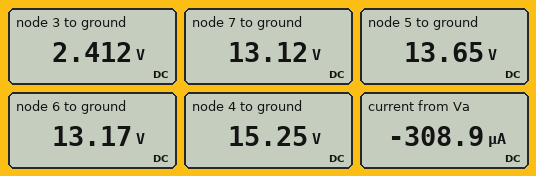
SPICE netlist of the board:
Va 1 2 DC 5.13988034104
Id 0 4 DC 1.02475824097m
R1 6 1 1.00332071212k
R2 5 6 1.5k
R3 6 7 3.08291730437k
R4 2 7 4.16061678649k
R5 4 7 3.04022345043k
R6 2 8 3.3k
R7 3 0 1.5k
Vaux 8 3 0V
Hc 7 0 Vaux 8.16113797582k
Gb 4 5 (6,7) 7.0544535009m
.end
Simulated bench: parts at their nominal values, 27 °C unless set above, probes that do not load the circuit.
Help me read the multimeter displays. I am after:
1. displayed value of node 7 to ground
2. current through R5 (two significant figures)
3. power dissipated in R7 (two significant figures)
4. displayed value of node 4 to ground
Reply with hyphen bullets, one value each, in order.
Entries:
- 13.12 V
- 700 µA
- 3.9 mW
- 15.25 V
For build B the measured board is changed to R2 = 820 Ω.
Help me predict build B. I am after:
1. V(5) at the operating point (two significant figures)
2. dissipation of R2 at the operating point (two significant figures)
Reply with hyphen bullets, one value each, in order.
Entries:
- 13 V
- 86 µW
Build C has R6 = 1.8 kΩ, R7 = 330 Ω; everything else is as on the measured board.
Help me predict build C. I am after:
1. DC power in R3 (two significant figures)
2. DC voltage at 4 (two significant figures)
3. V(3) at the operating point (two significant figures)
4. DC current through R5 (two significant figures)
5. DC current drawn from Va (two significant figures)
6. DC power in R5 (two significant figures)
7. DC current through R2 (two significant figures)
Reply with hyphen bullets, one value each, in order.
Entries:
- 930 nW
- 11 V
- 260 mV
- 1.4 mA
- 360 µA
- 6.0 mW
- 380 µA
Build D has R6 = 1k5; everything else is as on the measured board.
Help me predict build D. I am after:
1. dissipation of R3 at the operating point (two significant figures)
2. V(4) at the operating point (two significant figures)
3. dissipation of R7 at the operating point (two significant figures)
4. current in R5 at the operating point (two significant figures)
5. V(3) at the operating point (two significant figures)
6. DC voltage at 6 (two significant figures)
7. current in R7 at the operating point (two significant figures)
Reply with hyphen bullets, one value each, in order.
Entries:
- 380 nW
- 12 V
- 1.4 mW
- 1.3 mA
- 1.4 V
- 7.8 V
- 960 µA
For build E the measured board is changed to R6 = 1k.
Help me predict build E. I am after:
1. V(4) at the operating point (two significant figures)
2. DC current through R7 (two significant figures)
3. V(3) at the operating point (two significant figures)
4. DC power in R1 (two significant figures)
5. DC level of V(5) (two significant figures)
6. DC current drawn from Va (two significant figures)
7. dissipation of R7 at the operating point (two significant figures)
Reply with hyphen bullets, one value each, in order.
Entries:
- 11 V
- 860 µA
- 1.3 V
- 97 µW
- 6.5 V
- 310 µA
- 1.1 mW
